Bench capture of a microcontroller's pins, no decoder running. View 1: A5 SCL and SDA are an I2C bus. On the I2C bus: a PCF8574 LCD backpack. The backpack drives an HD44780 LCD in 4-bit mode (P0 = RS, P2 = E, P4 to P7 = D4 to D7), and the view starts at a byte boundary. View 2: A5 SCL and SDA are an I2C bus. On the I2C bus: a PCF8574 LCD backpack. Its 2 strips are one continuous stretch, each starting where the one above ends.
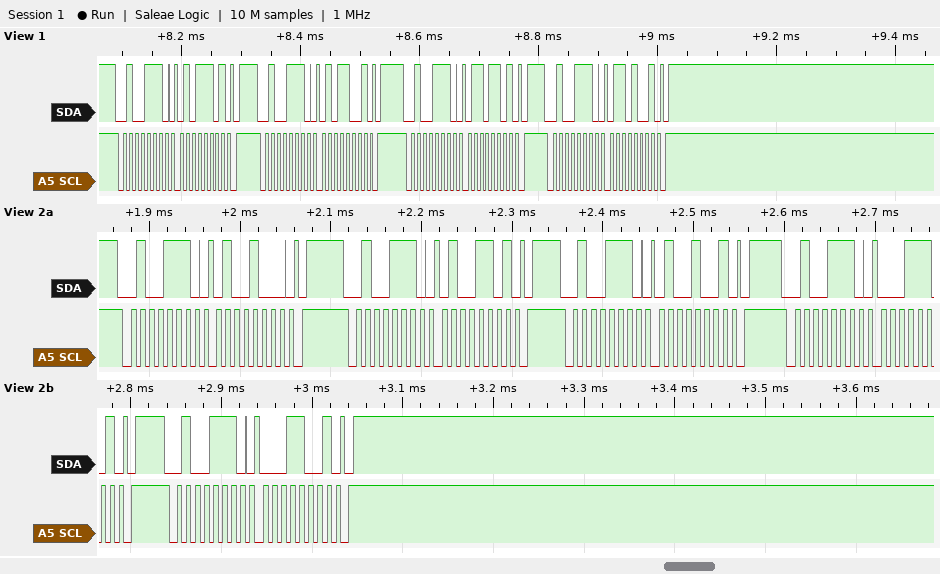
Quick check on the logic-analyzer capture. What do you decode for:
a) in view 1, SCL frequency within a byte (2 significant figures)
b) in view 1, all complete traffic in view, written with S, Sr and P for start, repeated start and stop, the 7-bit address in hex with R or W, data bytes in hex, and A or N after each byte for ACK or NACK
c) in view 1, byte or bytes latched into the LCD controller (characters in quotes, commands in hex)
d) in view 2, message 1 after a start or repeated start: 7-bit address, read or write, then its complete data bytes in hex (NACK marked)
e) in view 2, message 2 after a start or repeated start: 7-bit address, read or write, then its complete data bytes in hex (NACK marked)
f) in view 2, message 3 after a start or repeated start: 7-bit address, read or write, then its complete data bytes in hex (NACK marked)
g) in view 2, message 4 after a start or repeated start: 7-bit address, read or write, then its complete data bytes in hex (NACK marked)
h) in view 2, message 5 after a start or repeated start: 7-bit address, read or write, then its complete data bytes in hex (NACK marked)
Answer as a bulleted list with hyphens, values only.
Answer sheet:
- 100 kHz
- S 27W A 5D A P S 27W A 59 A P S 27W A 6D A P S 27W A 69 A P
- 'V'
- 0x27 write: 48
- 0x27 write: 4D
- 0x27 write: 49
- 0x27 write: 1D
- 0x27 write: 19
